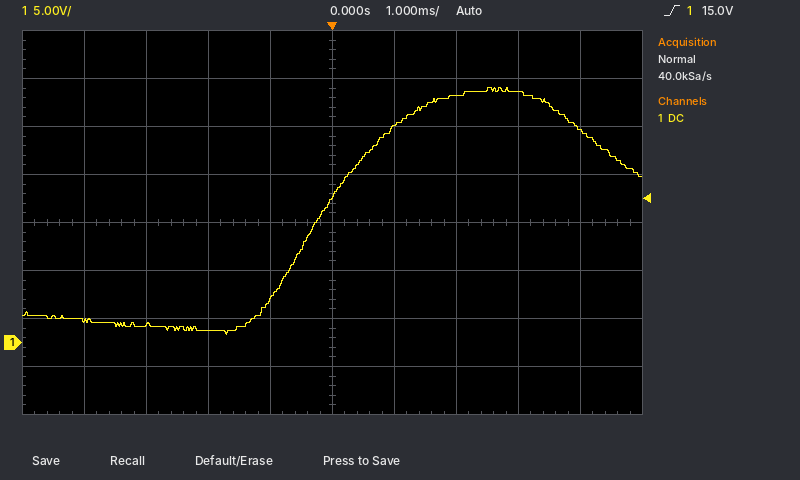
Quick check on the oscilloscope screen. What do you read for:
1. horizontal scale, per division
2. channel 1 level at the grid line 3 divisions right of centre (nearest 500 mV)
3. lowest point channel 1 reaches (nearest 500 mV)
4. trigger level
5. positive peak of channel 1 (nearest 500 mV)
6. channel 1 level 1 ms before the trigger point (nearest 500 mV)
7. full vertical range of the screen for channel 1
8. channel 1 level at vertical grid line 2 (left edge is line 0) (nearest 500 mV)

1 ms
26.0 V
1.0 V
15.0 V
26.5 V
4.5 V
40 V
2.0 V
